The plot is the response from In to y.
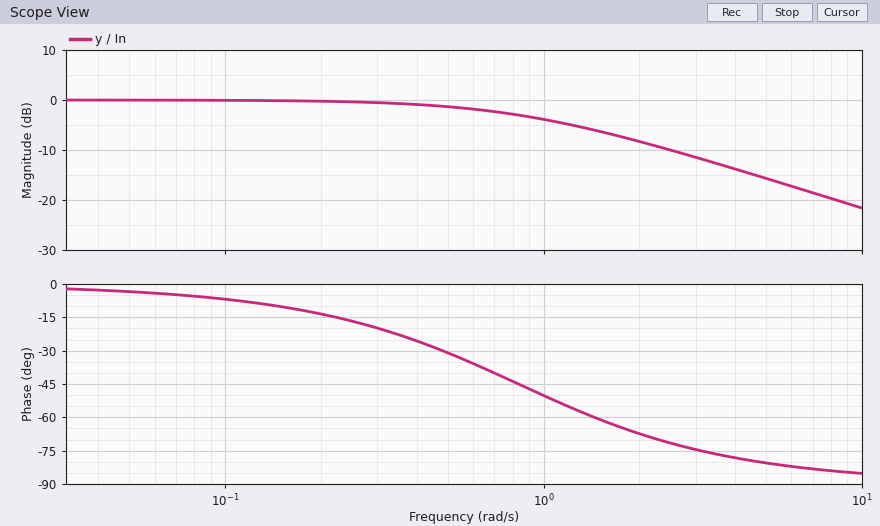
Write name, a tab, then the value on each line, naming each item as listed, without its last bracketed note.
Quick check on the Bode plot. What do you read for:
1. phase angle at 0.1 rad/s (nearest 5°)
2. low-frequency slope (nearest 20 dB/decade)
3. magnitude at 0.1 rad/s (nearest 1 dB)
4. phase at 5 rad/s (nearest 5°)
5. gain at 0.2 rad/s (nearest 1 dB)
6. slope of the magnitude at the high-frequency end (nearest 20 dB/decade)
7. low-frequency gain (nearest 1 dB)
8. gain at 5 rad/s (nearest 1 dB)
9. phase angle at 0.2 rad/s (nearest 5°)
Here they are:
phase angle at 0.1 rad/s	-5°
low-frequency slope	0 dB/decade
magnitude at 0.1 rad/s	0 dB
phase at 5 rad/s	-80°
gain at 0.2 rad/s	0 dB
slope of the magnitude at the high-frequency end	-20 dB/decade
low-frequency gain	0 dB
gain at 5 rad/s	-16 dB
phase angle at 0.2 rad/s	-15°
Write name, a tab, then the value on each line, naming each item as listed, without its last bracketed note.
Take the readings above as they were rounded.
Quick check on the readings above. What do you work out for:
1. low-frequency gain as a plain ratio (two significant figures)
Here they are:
low-frequency gain as a plain ratio	1.0
